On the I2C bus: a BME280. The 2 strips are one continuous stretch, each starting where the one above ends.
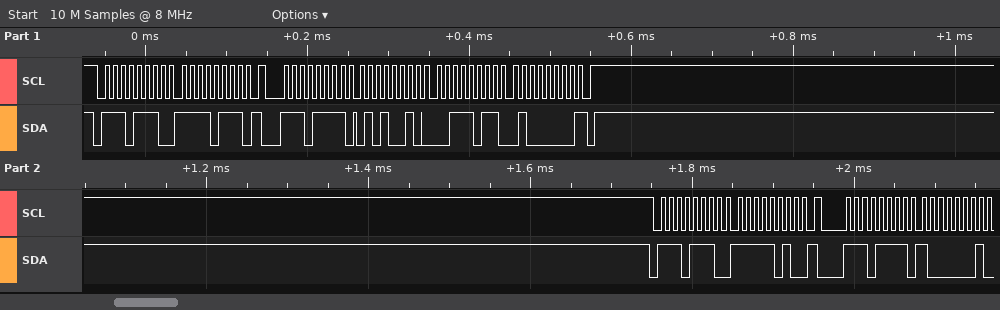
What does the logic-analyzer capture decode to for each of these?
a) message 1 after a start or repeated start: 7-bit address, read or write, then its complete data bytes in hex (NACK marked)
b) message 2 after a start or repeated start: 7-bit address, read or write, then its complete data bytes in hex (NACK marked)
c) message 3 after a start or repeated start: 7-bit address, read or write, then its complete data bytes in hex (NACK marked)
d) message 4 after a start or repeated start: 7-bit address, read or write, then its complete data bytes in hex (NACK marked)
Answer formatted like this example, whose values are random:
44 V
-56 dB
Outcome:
0x77 write: F7
0x77 read: 52 3B 40 NACK
0x77 write: FA
0x77 read: 81
